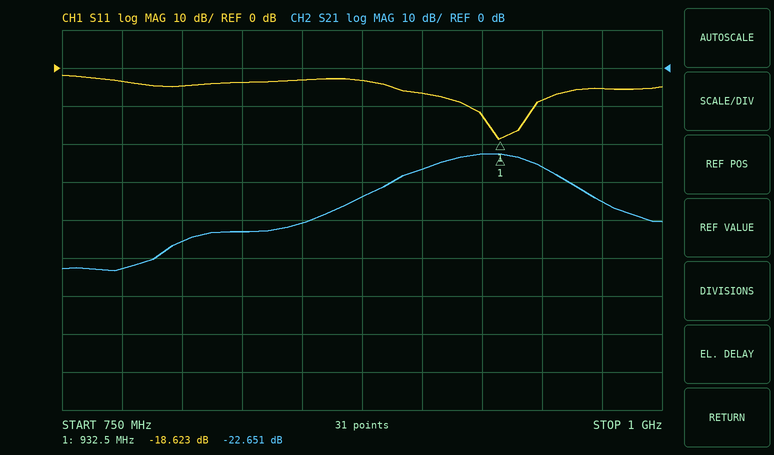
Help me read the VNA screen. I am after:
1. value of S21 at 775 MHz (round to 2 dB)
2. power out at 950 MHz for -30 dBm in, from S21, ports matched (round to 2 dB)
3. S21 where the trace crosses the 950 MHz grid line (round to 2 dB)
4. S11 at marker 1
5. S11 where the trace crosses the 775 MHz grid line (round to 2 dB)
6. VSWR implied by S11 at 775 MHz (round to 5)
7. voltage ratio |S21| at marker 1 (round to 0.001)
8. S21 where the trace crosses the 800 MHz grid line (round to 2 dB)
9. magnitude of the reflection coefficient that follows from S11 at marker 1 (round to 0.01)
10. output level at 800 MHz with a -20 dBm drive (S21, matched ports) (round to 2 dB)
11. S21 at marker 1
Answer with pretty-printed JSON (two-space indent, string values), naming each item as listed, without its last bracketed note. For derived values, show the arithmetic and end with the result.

{
  "value of S21 at 775 MHz": "-52 dB",
  "power out at 950 MHz for -30 dBm in, from S21, ports matched": "-30 dBm + (-26 dB) = -56 dBm",
  "S21 where the trace crosses the 950 MHz grid line": "-26 dB",
  "S11 at marker 1": "-18.623 dB",
  "S11 where the trace crosses the 775 MHz grid line": "-4 dB",
  "VSWR implied by S11 at 775 MHz": "|Γ| = 10^(-4/20) = 0.6310; VSWR = (1 + 0.6310)/(1 − 0.6310) ≈ 4.42, so 5 to the nearest 5",
  "voltage ratio |S21| at marker 1": "10^(-22.651/20) ≈ 0.074",
  "S21 where the trace crosses the 800 MHz grid line": "-46 dB",
  "magnitude of the reflection coefficient that follows from S11 at marker 1": "10^(-18.623/20) ≈ 0.12",
  "output level at 800 MHz with a -20 dBm drive (S21, matched ports)": "-20 dBm + (-46 dB) = -66 dBm",
  "S21 at marker 1": "-22.651 dB"
}
